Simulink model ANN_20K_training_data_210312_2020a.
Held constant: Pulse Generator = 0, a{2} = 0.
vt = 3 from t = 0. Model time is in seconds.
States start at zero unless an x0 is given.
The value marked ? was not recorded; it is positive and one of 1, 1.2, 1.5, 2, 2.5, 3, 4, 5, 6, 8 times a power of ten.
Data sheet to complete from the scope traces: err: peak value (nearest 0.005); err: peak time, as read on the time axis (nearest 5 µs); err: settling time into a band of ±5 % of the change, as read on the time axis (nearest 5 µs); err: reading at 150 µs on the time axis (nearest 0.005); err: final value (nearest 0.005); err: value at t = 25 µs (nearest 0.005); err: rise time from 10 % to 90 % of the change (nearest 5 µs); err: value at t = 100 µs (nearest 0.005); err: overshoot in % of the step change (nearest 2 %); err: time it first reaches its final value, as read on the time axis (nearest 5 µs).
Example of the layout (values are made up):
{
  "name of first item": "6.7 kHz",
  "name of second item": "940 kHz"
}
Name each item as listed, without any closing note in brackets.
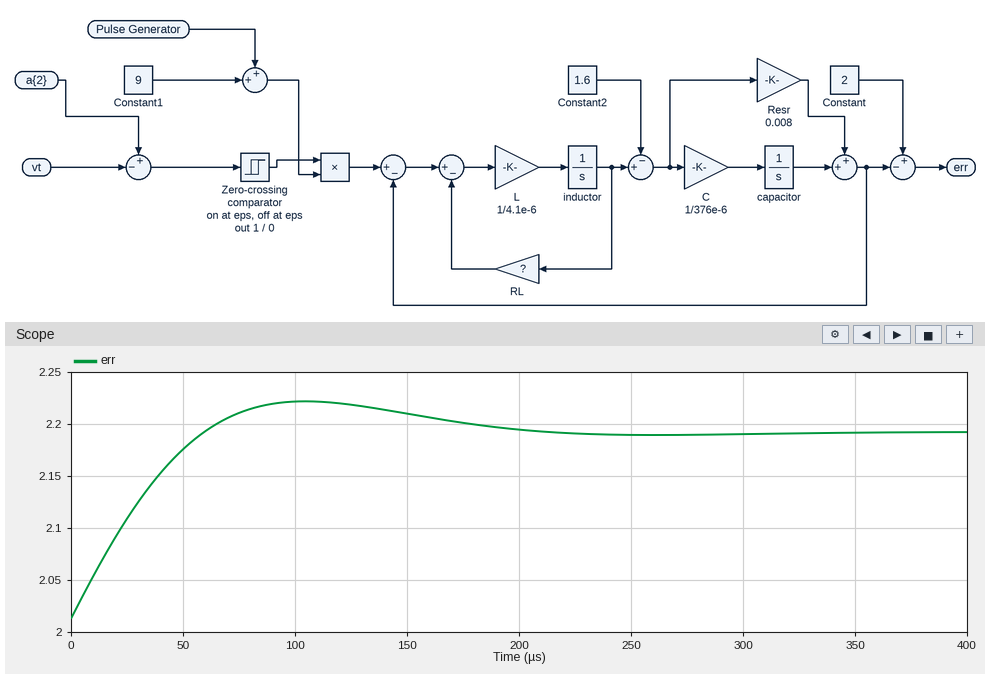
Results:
{
  "err: peak value": "2.220",
  "err: peak time, as read on the time axis": "105 µs",
  "err: settling time into a band of ±5 % of the change, as read on the time axis": "175 µs",
  "err: reading at 150 µs on the time axis": "2.210",
  "err: final value": "2.190",
  "err: value at t = 25 µs": "2.110",
  "err: rise time from 10 % to 90 % of the change": "45 µs",
  "err: value at t = 100 µs": "2.220",
  "err: overshoot in % of the step change": "16 %",
  "err: time it first reaches its final value, as read on the time axis": "60 µs"
}
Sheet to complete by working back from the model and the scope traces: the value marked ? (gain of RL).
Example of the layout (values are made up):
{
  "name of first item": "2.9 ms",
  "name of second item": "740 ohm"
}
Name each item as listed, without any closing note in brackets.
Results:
{
  "the value marked ?": "0.12"
}
